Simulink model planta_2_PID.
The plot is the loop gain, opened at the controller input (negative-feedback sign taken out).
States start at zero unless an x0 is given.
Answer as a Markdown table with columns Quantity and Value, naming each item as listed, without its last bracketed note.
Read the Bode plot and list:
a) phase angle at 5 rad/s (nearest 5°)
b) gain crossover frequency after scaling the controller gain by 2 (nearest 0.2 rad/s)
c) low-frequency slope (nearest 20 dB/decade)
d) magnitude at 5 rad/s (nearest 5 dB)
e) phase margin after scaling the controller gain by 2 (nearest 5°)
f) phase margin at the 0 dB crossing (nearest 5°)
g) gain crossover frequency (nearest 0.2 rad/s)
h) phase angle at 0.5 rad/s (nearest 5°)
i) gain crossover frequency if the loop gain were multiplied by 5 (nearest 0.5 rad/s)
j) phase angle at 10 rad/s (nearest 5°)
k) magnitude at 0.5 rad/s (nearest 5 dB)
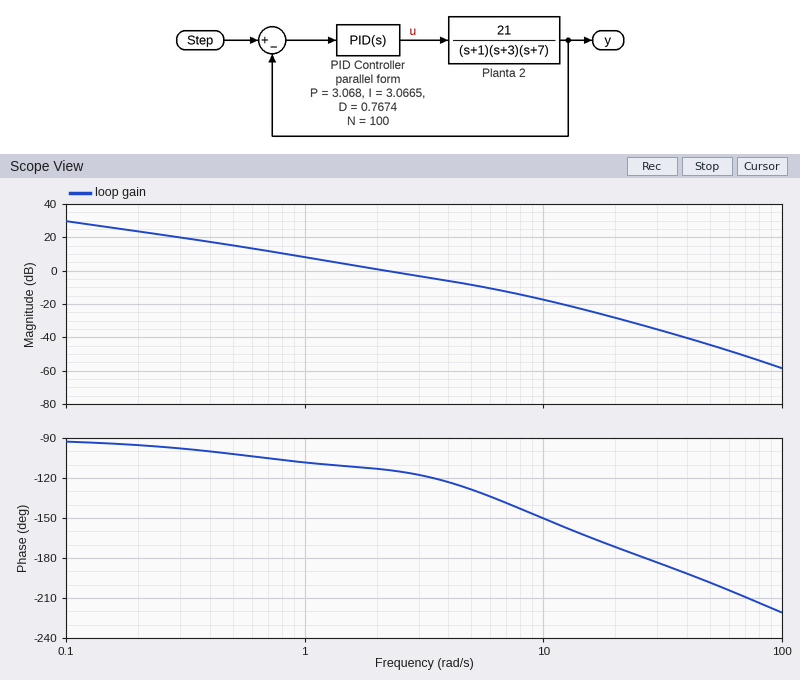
| Quantity | Value |
|---|---|
| phase angle at 5 rad/s | -130° |
| gain crossover frequency after scaling the controller gain by 2 | 4.0 rad/s |
| low-frequency slope | -20 dB/decade |
| magnitude at 5 rad/s | -10 dB |
| phase margin after scaling the controller gain by 2 | 55° |
| phase margin at the 0 dB crossing | 65° |
| gain crossover frequency | 2.2 rad/s |
| phase angle at 0.5 rad/s | -100° |
| gain crossover frequency if the loop gain were multiplied by 5 | 8.0 rad/s |
| phase angle at 10 rad/s | -150° |
| magnitude at 0.5 rad/s | 15 dB |
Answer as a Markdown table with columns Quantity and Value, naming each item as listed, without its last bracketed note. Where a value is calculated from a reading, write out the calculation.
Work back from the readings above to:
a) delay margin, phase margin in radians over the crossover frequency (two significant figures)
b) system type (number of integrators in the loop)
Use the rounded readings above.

| Quantity | Value |
|---|---|
| delay margin, phase margin in radians over the crossover frequency | 65 × π / 180 / 2.2 = 0.52 s |
| system type | 1 |
